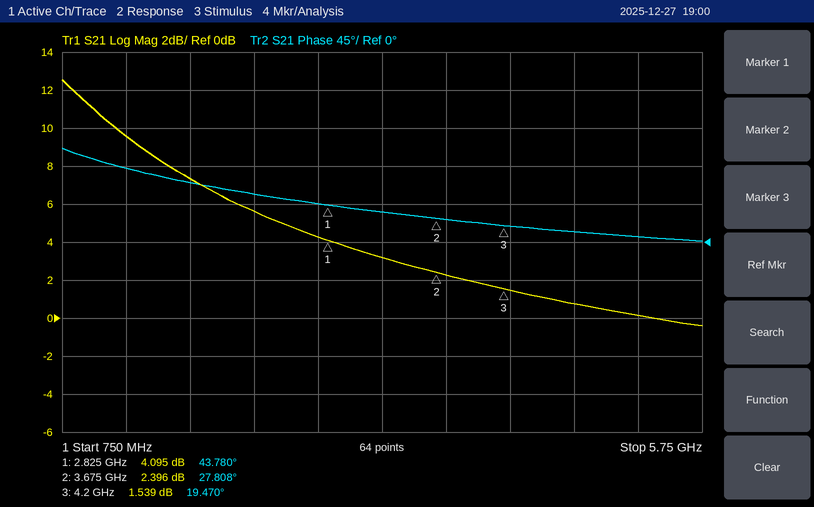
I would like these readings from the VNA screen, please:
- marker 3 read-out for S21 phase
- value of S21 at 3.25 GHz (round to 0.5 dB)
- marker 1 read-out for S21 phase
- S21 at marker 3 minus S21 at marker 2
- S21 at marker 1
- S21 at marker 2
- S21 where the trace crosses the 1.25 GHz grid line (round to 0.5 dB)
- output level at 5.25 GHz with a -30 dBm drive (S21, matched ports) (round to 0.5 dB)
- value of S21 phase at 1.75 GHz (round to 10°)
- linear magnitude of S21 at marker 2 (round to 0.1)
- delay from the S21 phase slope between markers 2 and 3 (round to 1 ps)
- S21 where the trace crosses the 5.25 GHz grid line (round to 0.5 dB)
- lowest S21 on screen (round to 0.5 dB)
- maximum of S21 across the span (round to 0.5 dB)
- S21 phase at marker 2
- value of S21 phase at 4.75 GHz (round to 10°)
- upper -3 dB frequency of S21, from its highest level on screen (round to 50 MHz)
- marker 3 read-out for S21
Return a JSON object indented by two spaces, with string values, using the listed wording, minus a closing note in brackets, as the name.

{
  "marker 3 read-out for S21 phase": "19.470°",
  "value of S21 at 3.25 GHz": "3.0 dB",
  "marker 1 read-out for S21 phase": "43.780°",
  "S21 at marker 3 minus S21 at marker 2": "-0.857 dB",
  "S21 at marker 1": "4.095 dB",
  "S21 at marker 2": "2.396 dB",
  "S21 where the trace crosses the 1.25 GHz grid line": "9.5 dB",
  "output level at 5.25 GHz with a -30 dBm drive (S21, matched ports)": "-30.0 dBm",
  "value of S21 phase at 1.75 GHz": "70°",
  "linear magnitude of S21 at marker 2": "1.3",
  "delay from the S21 phase slope between markers 2 and 3": "44 ps",
  "S21 where the trace crosses the 5.25 GHz grid line": "0.0 dB",
  "lowest S21 on screen": "-0.5 dB",
  "maximum of S21 across the span": "12.5 dB",
  "S21 phase at marker 2": "27.808°",
  "value of S21 phase at 4.75 GHz": "10°",
  "upper -3 dB frequency of S21, from its highest level on screen": "1.25 GHz",
  "marker 3 read-out for S21": "1.539 dB"
}
